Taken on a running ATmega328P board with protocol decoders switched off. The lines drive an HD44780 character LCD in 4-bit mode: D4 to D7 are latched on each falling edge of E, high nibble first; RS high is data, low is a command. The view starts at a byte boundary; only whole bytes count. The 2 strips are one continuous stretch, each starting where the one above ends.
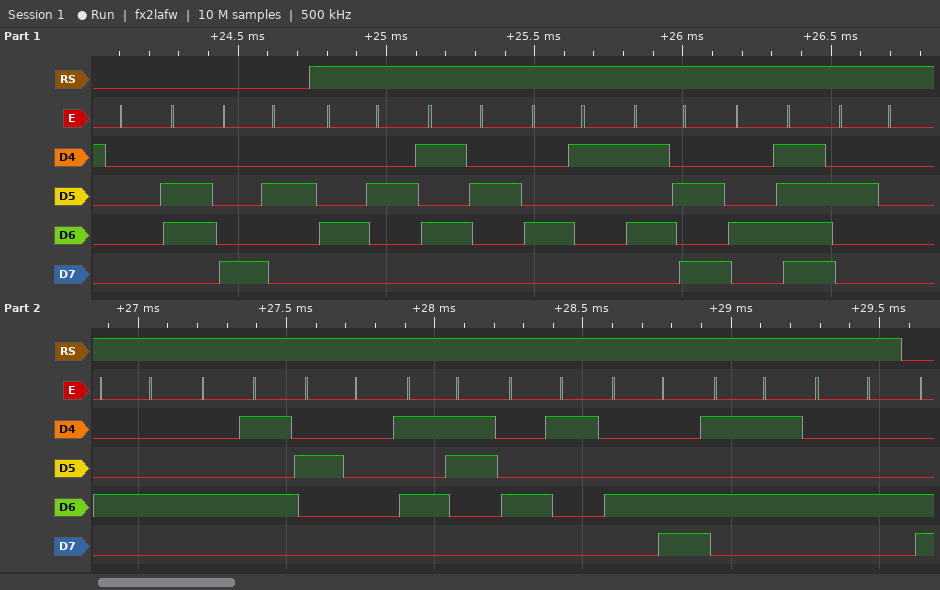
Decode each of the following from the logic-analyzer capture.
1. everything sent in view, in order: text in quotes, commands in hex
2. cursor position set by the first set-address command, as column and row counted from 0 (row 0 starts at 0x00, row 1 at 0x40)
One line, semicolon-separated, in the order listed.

0x06 0x82 "BRAZO DE SALUD"; column 2, row 0
